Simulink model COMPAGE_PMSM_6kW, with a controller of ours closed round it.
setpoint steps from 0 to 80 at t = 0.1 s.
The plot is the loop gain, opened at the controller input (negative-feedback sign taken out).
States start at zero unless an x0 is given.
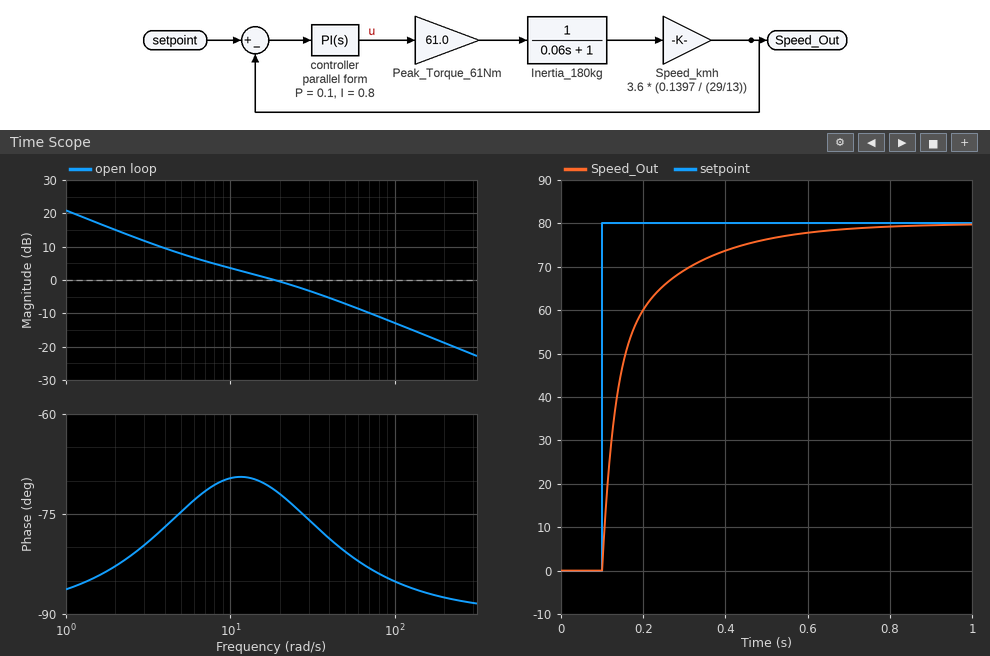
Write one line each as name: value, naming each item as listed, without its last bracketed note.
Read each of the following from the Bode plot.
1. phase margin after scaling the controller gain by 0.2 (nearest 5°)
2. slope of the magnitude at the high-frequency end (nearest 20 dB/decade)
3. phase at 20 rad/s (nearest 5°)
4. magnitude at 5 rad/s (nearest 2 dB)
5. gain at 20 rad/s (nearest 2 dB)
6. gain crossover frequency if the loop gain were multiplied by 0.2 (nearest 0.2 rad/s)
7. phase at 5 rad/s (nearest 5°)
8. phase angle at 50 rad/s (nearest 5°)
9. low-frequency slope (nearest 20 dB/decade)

phase margin after scaling the controller gain by 0.2: 100°
slope of the magnitude at the high-frequency end: -20 dB/decade
phase at 20 rad/s: -70°
magnitude at 5 rad/s: 8 dB
gain at 20 rad/s: 0 dB
gain crossover frequency if the loop gain were multiplied by 0.2: 2.2 rad/s
phase at 5 rad/s: -75°
phase angle at 50 rad/s: -80°
low-frequency slope: -20 dB/decade
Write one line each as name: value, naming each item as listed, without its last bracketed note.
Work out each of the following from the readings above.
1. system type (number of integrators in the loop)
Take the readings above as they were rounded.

system type: 1
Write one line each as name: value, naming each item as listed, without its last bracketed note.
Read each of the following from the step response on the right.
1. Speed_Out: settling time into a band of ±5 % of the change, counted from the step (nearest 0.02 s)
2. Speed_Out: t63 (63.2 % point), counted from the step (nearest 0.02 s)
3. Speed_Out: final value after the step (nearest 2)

Speed_Out: settling time into a band of ±5 % of the change, counted from the step: 0.38 s
Speed_Out: t63 (63.2 % point), counted from the step: 0.06 s
Speed_Out: final value after the step: 80
